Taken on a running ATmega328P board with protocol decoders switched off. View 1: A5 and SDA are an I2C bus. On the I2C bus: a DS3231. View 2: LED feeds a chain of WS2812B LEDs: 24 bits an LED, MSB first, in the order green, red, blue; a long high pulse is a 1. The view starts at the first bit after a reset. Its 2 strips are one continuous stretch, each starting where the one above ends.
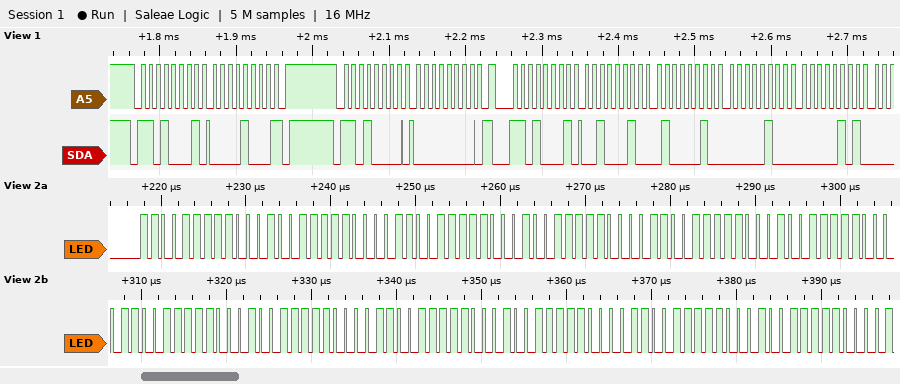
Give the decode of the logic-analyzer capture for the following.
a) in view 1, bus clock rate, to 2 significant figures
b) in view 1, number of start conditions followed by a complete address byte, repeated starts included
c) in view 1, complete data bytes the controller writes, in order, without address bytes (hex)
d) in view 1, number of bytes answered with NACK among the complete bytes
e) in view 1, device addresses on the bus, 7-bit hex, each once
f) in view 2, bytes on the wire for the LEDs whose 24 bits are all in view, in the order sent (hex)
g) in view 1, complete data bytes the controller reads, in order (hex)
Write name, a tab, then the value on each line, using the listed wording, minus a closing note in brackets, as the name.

in view 1, bus clock rate, to 2 significant figures	100 kHz
in view 1, number of start conditions followed by a complete address byte, repeated starts included	3
in view 1, complete data bytes the controller writes, in order, without address bytes	00
in view 1, number of bytes answered with NACK among the complete bytes	1
in view 1, device addresses on the bus, 7-bit hex, each once	0x68
in view 2, bytes on the wire for the LEDs whose 24 bits are all in view, in the order sent	CF 89 F0 CF 89 F0 CF 89 F0 CF 89 F0 CF 89 F0 CF 89 F0
in view 1, complete data bytes the controller reads, in order	08 22 42 04 05
